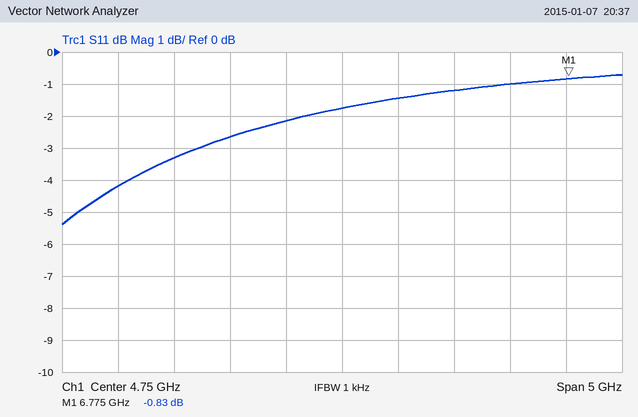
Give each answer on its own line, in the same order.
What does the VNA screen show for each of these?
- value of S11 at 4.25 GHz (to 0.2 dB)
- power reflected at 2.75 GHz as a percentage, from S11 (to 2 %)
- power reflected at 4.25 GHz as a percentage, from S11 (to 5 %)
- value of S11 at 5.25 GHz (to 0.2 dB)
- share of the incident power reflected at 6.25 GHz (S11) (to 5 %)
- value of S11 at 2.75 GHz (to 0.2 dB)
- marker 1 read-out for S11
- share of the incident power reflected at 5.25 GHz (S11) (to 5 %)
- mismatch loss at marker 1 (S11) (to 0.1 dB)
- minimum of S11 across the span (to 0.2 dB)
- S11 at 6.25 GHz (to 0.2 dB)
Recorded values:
-2.2 dB
38 %
60 %
-1.4 dB
80 %
-4.2 dB
-0.83 dB
70 %
7.6 dB
-5.4 dB
-1.0 dB
